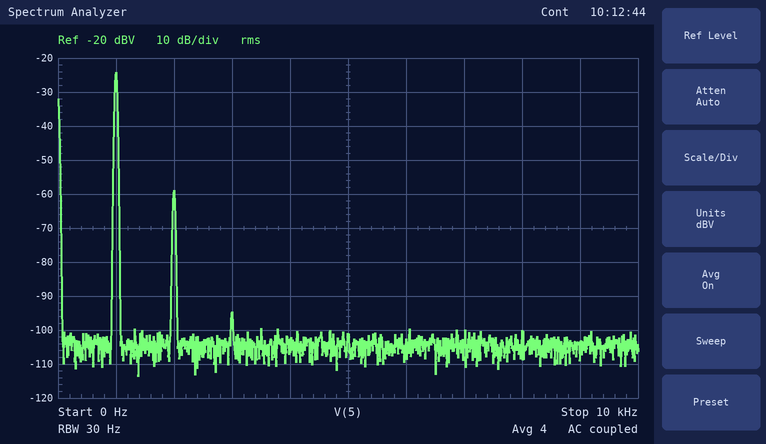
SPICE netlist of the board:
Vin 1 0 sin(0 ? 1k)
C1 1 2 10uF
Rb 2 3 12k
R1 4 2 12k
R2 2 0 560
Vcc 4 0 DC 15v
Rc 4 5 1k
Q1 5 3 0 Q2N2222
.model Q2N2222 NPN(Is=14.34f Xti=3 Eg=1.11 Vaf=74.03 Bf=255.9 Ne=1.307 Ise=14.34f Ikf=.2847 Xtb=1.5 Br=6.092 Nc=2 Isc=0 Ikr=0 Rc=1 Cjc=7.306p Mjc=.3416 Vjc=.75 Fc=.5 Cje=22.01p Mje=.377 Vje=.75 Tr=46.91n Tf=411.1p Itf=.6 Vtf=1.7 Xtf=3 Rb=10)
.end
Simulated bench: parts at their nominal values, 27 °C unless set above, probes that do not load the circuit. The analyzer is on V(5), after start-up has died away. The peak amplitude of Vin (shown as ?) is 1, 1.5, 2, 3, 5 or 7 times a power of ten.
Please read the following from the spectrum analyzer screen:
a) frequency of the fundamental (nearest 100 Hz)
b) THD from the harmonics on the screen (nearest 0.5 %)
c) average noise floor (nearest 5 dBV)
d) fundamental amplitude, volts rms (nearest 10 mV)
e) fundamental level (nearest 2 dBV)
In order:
1.0 kHz
2.0 %
-105 dBV
60 mV
-24 dBV
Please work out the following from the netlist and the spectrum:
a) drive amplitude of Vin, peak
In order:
10 mV
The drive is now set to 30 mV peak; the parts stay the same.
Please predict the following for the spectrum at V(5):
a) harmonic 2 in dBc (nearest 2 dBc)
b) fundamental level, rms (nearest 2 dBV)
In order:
-26 dBc
-14 dBV
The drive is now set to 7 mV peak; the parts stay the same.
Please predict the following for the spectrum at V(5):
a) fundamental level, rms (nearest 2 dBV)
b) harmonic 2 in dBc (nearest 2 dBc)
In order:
-28 dBV
-38 dBc
